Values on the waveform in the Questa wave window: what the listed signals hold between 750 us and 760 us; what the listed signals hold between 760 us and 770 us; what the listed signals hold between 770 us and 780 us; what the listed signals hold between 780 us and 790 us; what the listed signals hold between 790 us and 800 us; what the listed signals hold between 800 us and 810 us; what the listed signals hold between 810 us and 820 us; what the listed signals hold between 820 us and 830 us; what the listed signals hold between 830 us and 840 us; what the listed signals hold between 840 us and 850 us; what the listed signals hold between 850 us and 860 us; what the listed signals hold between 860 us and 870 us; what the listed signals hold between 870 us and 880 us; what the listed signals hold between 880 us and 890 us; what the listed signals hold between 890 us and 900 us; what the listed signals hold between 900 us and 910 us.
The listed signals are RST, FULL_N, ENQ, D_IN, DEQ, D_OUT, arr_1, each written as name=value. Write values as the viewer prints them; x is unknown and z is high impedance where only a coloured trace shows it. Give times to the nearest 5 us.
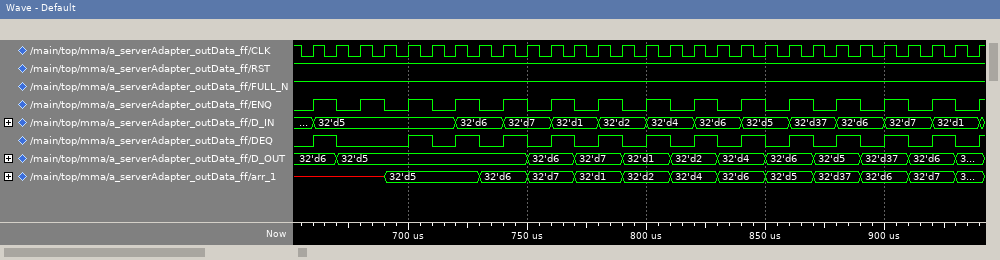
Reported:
RST=1, FULL_N=1, ENQ=0, D_IN=32'd7, DEQ=0, D_OUT=32'd6, arr_1=32'd7
RST=1, FULL_N=1, ENQ=1, D_IN=32'd1, DEQ=1, D_OUT=32'd6, arr_1=32'd7
RST=1, FULL_N=1, ENQ=0, D_IN=32'd1, DEQ=0, D_OUT=32'd7, arr_1=32'd1
RST=1, FULL_N=1, ENQ=1, D_IN=32'd2, DEQ=1, D_OUT=32'd7, arr_1=32'd1
RST=1, FULL_N=1, ENQ=0, D_IN=32'd2, DEQ=0, D_OUT=32'd1, arr_1=32'd2
RST=1, FULL_N=1, ENQ=1, D_IN=32'd4, DEQ=1, D_OUT=32'd1, arr_1=32'd2
RST=1, FULL_N=1, ENQ=0, D_IN=32'd4, DEQ=0, D_OUT=32'd2, arr_1=32'd4
RST=1, FULL_N=1, ENQ=1, D_IN=32'd6, DEQ=1, D_OUT=32'd2, arr_1=32'd4
RST=1, FULL_N=1, ENQ=0, D_IN=32'd6, DEQ=0, D_OUT=32'd4, arr_1=32'd6
RST=1, FULL_N=1, ENQ=1, D_IN=32'd5, DEQ=1, D_OUT=32'd4, arr_1=32'd6
RST=1, FULL_N=1, ENQ=0, D_IN=32'd5, DEQ=0, D_OUT=32'd6, arr_1=32'd5
RST=1, FULL_N=1, ENQ=1, D_IN=32'd37, DEQ=1, D_OUT=32'd6, arr_1=32'd5
RST=1, FULL_N=1, ENQ=0, D_IN=32'd37, DEQ=0, D_OUT=32'd5, arr_1=32'd37
RST=1, FULL_N=1, ENQ=1, D_IN=32'd6, DEQ=1, D_OUT=32'd5, arr_1=32'd37
RST=1, FULL_N=1, ENQ=0, D_IN=32'd6, DEQ=0, D_OUT=32'd37, arr_1=32'd6
RST=1, FULL_N=1, ENQ=1, D_IN=32'd7, DEQ=1, D_OUT=32'd37, arr_1=32'd6
